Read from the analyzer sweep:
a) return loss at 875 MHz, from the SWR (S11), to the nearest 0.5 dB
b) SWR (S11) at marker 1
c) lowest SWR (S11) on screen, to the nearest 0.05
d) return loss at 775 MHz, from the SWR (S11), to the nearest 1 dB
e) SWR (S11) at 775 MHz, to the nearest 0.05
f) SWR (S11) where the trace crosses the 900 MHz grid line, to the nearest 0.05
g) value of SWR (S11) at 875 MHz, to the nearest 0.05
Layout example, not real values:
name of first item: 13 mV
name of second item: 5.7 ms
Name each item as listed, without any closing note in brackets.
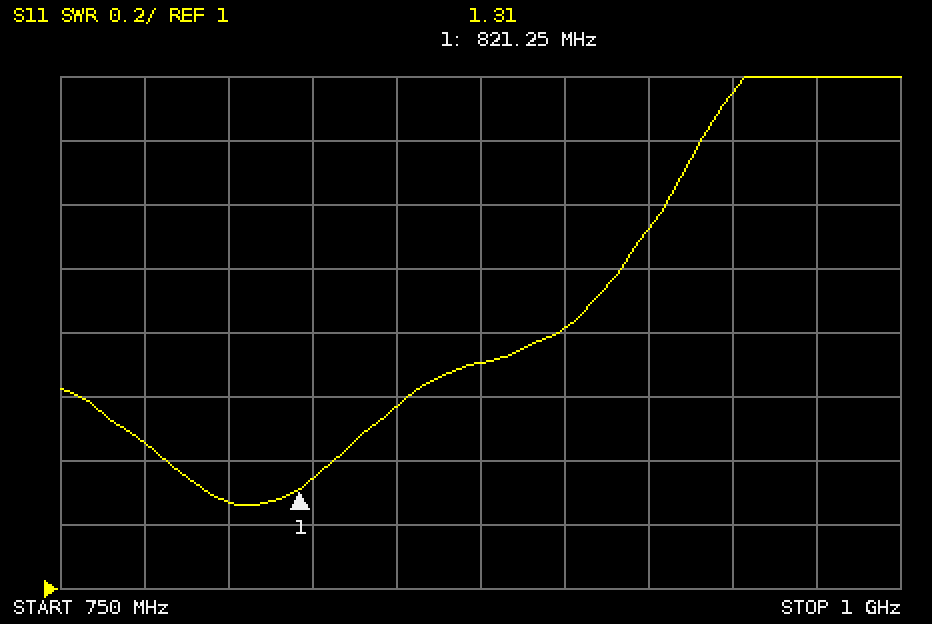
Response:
return loss at 875 MHz, from the SWR (S11), to the nearest 0.5 dB: 11.5 dB
SWR (S11) at marker 1: 1.31
lowest SWR (S11) on screen, to the nearest 0.05: 1.25
return loss at 775 MHz, from the SWR (S11), to the nearest 1 dB: 15 dB
SWR (S11) at 775 MHz, to the nearest 0.05: 1.45
SWR (S11) where the trace crosses the 900 MHz grid line, to the nearest 0.05: 1.80
value of SWR (S11) at 875 MHz, to the nearest 0.05: 1.70
